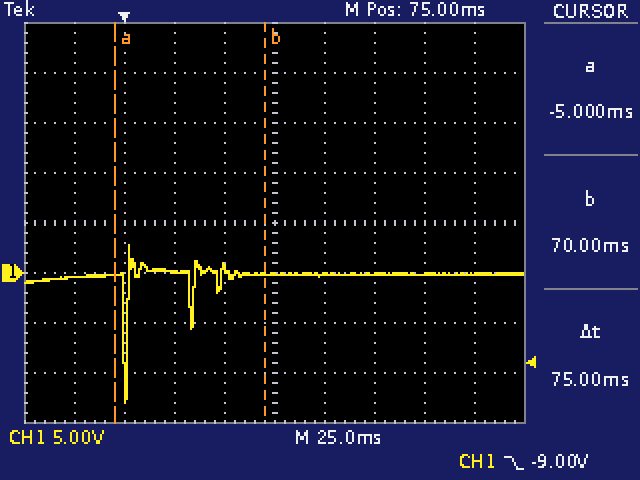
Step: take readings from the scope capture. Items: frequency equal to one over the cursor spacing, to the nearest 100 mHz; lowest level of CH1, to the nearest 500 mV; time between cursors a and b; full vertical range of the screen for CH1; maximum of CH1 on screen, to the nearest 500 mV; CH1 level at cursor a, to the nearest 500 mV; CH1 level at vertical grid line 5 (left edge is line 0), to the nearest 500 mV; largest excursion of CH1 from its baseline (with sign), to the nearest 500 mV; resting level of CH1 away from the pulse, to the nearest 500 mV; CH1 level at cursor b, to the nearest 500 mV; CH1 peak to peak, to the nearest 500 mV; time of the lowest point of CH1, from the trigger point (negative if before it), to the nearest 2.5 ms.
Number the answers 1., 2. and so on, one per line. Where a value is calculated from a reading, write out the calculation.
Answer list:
1. 1 / 75 ms ≈ 13.3 Hz
2. -13.0 V
3. 75 ms
4. 40 V
5. 3.0 V
6. 0.0 V
7. 0.0 V
8. -13.0 V − (0.0 V) = -13.0 V
9. 0.0 V
10. 0.0 V
11. 3.0 V − (-13.0 V) = 16.0 V
12. 0.0 ms
